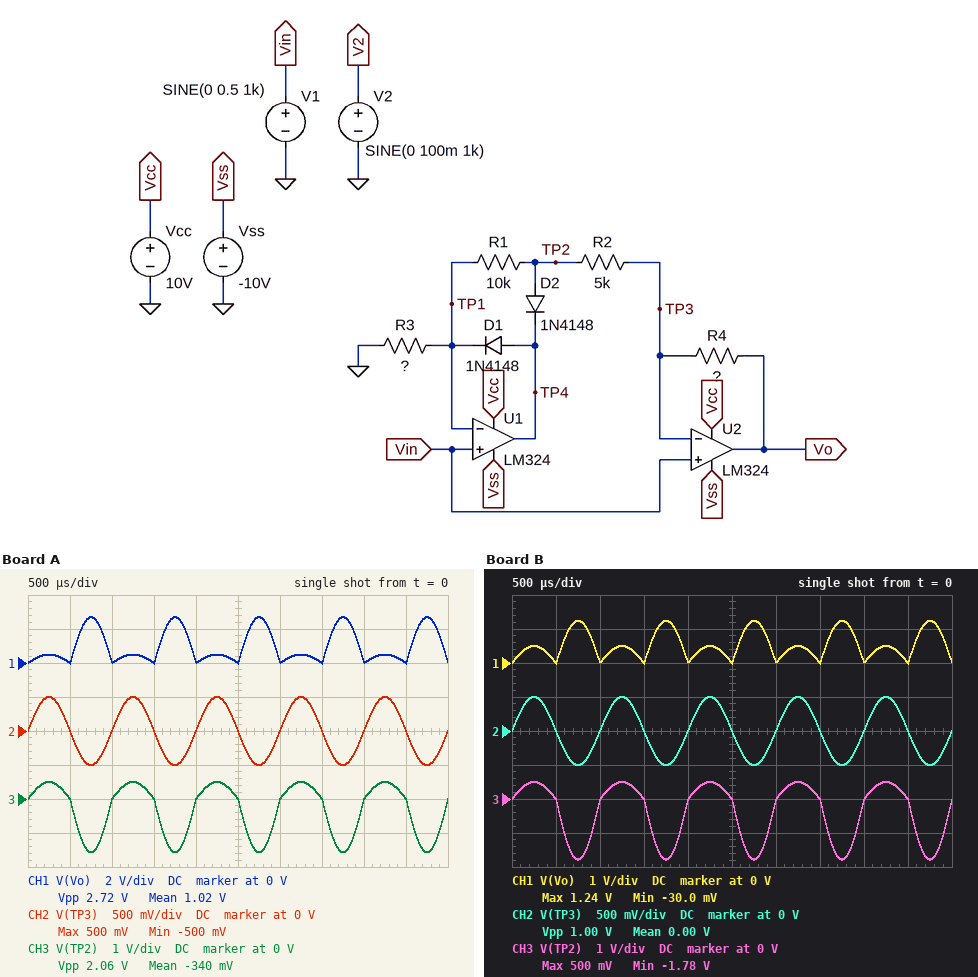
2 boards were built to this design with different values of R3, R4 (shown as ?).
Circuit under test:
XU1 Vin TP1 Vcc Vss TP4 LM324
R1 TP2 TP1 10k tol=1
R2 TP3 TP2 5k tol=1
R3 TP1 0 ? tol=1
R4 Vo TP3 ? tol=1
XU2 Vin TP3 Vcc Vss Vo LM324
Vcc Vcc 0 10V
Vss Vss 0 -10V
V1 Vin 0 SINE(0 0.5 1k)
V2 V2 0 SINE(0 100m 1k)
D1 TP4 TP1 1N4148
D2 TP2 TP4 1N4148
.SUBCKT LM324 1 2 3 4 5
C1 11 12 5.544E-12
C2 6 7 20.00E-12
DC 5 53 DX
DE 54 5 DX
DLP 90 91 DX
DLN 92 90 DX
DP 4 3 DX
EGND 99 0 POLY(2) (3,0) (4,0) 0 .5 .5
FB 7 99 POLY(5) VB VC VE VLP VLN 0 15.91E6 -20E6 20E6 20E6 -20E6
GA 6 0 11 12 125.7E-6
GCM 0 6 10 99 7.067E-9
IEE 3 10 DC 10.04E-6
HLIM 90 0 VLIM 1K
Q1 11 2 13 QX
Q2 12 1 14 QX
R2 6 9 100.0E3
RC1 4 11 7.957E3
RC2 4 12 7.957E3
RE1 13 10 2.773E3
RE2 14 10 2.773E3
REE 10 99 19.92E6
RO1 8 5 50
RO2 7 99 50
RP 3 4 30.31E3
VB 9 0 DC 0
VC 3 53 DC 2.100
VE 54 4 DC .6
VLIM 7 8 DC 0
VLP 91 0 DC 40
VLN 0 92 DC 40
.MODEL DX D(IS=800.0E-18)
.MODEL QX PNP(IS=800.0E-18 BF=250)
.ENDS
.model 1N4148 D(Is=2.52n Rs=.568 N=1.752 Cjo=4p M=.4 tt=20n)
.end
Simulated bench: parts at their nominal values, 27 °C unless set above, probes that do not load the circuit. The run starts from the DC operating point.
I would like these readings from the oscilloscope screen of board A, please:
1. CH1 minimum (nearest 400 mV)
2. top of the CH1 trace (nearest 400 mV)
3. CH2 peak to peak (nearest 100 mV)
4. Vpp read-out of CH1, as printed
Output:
0 V
2.8 V
1.0 V
2.72 V
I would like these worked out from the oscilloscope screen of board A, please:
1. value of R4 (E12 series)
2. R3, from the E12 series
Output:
15 kΩ
4.7 kΩ
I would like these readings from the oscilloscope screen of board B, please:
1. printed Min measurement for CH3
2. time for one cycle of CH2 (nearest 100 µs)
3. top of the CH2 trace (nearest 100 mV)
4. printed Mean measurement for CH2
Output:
-1.78 V
1.0 ms
500 mV
0.00 V
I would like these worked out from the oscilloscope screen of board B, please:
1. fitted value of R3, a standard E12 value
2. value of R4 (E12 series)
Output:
3.9 kΩ
6.8 kΩ
